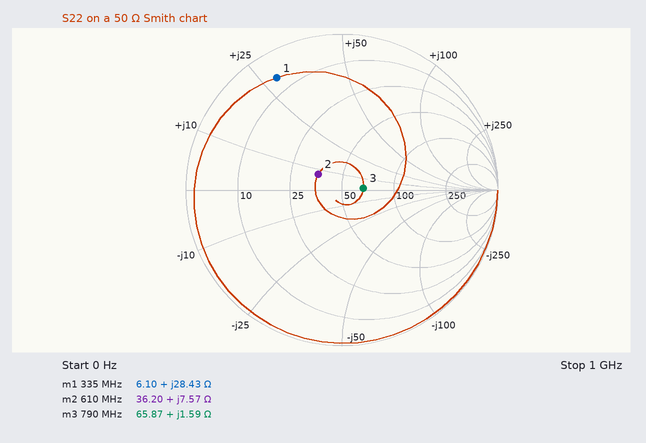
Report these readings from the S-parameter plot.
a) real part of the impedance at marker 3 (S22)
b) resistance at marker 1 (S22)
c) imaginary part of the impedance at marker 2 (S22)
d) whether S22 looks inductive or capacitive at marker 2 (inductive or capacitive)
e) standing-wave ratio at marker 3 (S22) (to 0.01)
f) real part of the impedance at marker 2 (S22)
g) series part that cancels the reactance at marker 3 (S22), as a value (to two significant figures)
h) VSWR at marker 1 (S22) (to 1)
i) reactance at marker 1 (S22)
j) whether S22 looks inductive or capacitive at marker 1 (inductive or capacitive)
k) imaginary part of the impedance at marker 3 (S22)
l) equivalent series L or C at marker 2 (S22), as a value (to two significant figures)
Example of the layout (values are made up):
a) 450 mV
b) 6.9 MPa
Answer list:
a) 65.87 Ω
b) 6.10 Ω
c) +7.57 Ω
d) inductive
e) 1.32
f) 36.20 Ω
g) 130 pF
h) 11
i) +28.43 Ω
j) inductive
k) +1.59 Ω
l) 2.0 nH
